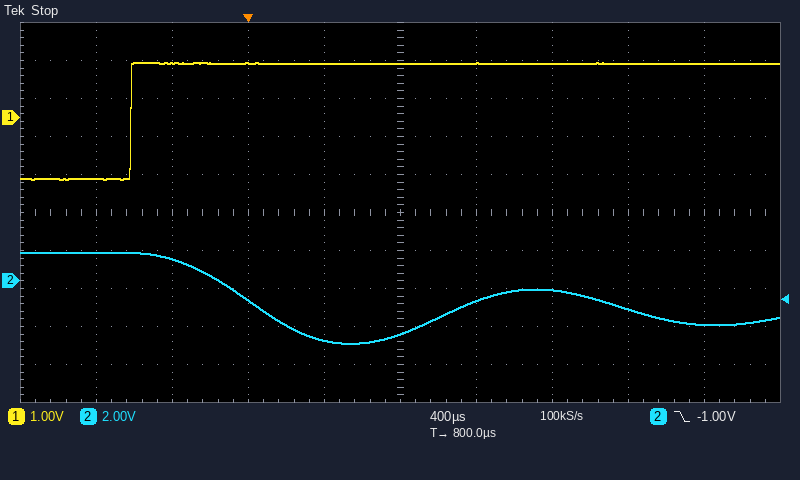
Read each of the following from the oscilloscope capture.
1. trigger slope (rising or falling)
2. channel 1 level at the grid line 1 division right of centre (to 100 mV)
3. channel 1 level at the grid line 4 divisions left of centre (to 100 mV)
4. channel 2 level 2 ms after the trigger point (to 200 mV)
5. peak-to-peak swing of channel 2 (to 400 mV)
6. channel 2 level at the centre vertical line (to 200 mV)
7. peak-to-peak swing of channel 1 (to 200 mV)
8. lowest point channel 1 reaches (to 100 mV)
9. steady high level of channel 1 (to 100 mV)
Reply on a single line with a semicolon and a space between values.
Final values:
falling; 1.4 V; -1.6 V; -1.4 V; 4.8 V; -2.8 V; 3.0 V; -1.6 V; 1.4 V
